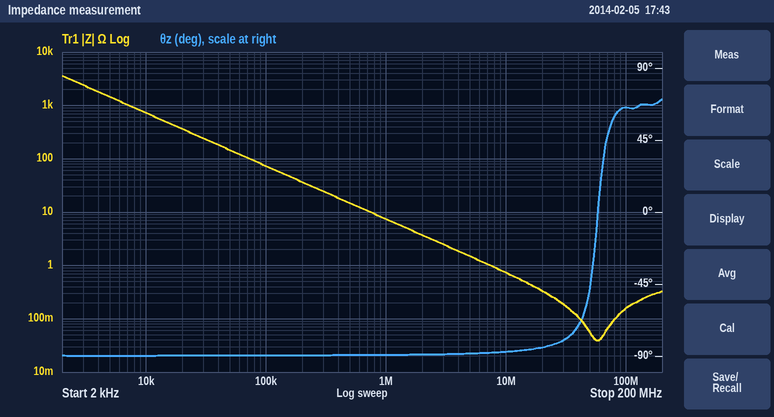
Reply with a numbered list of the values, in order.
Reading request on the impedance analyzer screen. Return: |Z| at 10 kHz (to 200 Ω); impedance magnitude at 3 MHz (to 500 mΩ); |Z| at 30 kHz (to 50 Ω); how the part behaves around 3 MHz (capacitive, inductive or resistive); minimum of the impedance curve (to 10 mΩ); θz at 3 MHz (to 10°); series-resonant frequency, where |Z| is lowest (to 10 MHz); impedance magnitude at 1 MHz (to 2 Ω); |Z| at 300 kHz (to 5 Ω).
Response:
1. 800 Ω
2. 2.5 Ω
3. 250 Ω
4. capacitive
5. 40 mΩ
6. -90°
7. 60 MHz
8. 8 Ω
9. 25 Ω
